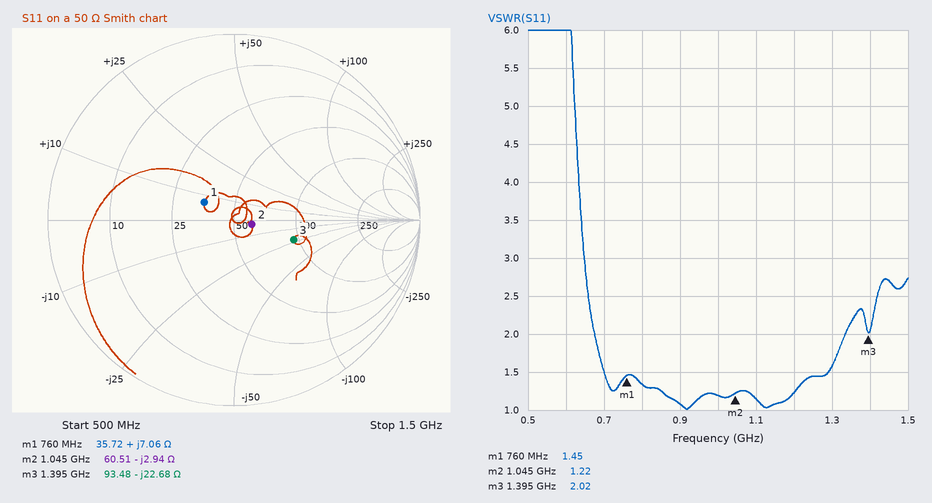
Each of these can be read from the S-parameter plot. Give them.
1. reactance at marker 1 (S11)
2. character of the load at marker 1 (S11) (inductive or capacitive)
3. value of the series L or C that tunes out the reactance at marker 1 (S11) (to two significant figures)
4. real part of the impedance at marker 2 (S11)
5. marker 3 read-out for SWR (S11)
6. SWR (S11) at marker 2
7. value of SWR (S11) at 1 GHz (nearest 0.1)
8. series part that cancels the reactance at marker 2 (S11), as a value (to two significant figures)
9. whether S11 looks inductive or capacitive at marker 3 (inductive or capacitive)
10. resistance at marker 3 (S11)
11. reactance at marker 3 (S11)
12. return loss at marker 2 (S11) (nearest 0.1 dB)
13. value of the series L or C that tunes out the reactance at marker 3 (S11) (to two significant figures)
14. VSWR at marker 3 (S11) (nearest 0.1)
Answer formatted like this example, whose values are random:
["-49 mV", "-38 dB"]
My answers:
["+7.06 Ω", "inductive", "30 pF", "60.51 Ω", "2.02", "1.22", "1.2", "450 pH", "capacitive", "93.48 Ω", "-22.68 Ω", "20.1 dB", "2.6 nH", "2.0"]
